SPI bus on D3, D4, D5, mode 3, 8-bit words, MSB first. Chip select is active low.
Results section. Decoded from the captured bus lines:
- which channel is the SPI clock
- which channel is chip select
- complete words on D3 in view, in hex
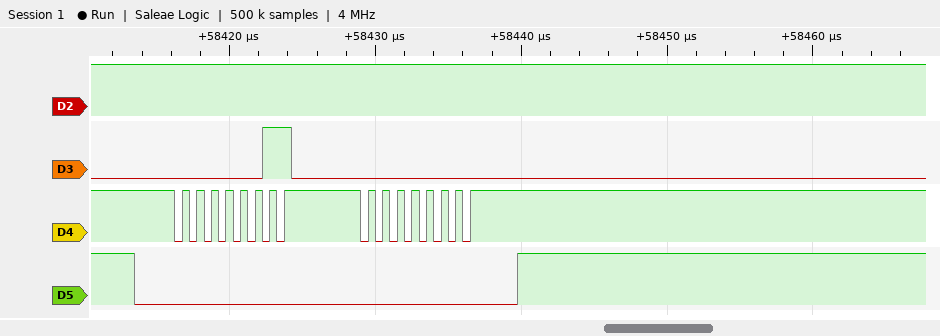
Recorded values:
D4
D5
03, 00
